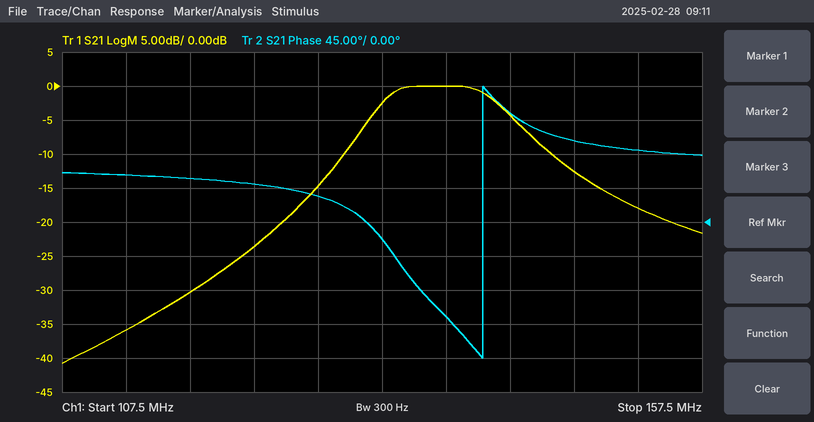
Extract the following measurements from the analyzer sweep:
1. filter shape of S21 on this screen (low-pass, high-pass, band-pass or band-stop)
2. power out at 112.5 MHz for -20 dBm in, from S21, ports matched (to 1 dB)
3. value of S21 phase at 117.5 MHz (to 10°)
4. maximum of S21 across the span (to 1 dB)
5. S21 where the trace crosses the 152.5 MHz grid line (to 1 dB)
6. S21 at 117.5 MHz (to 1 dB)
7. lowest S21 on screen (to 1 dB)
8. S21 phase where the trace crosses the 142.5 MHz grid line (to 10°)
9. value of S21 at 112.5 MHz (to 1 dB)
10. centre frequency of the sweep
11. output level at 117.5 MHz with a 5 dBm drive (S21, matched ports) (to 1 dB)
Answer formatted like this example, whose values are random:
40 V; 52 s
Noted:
band-pass; -56 dBm; 60°; 0 dB; -18 dB; -30 dB; -41 dB; 140°; -36 dB; 132.5 MHz; -25 dBm
